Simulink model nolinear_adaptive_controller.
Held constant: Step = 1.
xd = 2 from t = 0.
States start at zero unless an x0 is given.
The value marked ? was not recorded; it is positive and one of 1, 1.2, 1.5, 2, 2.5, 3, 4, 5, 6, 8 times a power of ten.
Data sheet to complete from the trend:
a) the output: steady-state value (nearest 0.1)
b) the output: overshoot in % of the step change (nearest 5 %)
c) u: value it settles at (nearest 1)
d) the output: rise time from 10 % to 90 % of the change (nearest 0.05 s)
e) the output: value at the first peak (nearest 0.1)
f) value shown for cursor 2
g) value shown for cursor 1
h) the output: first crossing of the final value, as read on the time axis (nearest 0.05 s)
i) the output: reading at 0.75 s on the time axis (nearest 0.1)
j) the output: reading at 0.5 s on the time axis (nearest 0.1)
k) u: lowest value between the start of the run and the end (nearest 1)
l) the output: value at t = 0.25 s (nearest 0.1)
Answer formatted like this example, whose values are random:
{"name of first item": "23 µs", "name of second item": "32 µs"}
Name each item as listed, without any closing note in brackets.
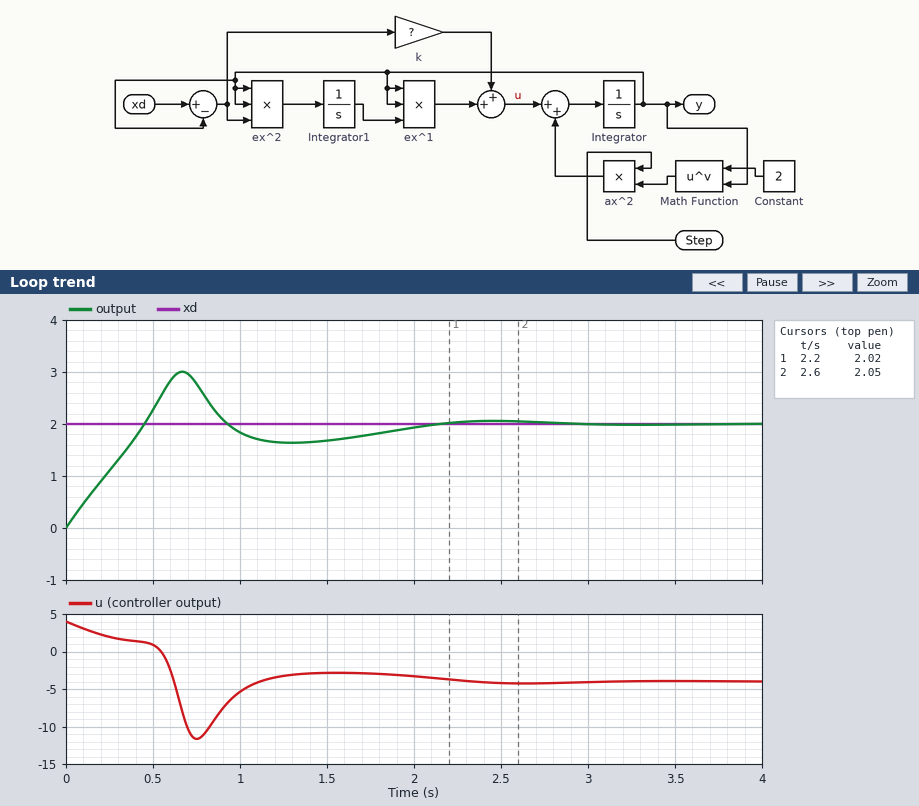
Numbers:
{"the output: steady-state value": "2.0", "the output: overshoot in % of the step change": "50 %", "u: value it settles at": "-4", "the output: rise time from 10 % to 90 % of the change": "0.35 s", "the output: value at the first peak": "3.0", "value shown for cursor 2": "2.05", "value shown for cursor 1": "2.02", "the output: first crossing of the final value, as read on the time axis": "0.45 s", "the output: reading at 0.75 s on the time axis": "2.8", "the output: reading at 0.5 s on the time axis": "2.3", "u: lowest value between the start of the run and the end": "-12", "the output: value at t = 0.25 s": "1.1"}
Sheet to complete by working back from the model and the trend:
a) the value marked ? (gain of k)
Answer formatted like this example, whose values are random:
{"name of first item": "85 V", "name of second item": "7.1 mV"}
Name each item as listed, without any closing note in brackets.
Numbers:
{"the value marked ?": "2"}
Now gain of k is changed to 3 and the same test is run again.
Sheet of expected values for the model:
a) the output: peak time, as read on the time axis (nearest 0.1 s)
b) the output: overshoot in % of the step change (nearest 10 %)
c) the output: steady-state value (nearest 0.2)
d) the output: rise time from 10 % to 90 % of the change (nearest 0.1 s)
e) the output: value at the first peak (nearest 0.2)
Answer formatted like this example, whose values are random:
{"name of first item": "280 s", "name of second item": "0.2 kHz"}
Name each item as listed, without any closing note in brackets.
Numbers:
{"the output: peak time, as read on the time axis": "0.6 s", "the output: overshoot in % of the step change": "40 %", "the output: steady-state value": "2.0", "the output: rise time from 10 % to 90 % of the change": "0.3 s", "the output: value at the first peak": "2.8"}
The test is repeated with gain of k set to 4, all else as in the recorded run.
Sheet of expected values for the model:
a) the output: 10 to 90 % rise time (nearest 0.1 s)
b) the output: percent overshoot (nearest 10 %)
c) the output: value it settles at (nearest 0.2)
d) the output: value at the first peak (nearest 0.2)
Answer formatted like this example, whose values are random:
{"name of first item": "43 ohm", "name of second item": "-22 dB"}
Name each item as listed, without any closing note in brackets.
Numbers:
{"the output: 10 to 90 % rise time": "0.3 s", "the output: percent overshoot": "40 %", "the output: value it settles at": "2.0", "the output: value at the first peak": "2.8"}
